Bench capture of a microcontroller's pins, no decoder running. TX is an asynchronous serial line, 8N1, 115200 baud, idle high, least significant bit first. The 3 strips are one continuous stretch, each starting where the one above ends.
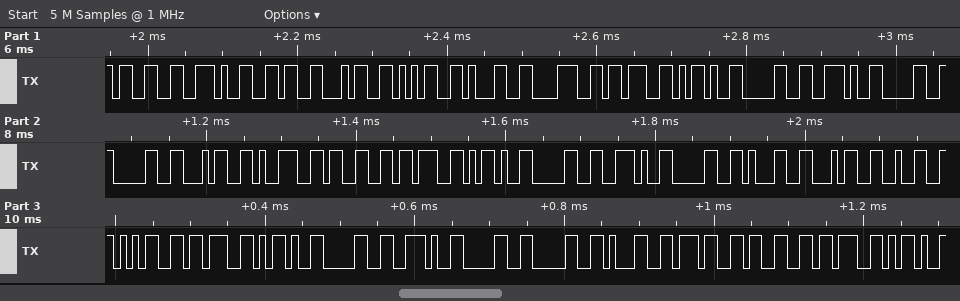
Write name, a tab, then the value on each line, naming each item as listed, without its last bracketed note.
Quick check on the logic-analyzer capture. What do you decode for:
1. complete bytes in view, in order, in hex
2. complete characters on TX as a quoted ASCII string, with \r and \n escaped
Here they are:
complete bytes in view, in order, in hex	33 2E 36 34 35 31 38 3B 2D 30 2E 30 30 34 39 33 3B 2D 30 2E 30 31 34 32 35 3B 2D 30 2E 30 30 31 37 33 3B 2D
complete characters on TX as a quoted ASCII string, with \r and \n escaped	"3.64518;-0.00493;-0.01425;-0.00173;-"
